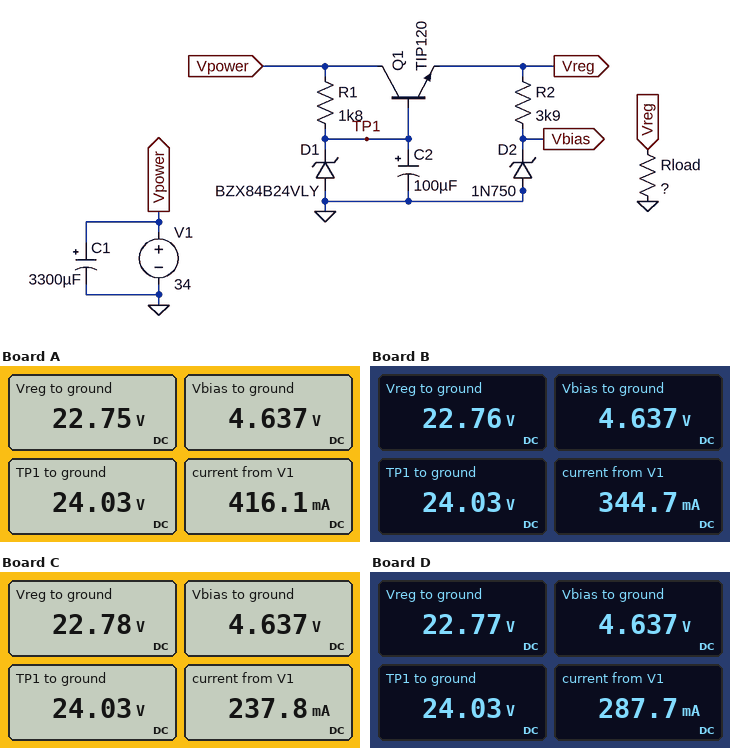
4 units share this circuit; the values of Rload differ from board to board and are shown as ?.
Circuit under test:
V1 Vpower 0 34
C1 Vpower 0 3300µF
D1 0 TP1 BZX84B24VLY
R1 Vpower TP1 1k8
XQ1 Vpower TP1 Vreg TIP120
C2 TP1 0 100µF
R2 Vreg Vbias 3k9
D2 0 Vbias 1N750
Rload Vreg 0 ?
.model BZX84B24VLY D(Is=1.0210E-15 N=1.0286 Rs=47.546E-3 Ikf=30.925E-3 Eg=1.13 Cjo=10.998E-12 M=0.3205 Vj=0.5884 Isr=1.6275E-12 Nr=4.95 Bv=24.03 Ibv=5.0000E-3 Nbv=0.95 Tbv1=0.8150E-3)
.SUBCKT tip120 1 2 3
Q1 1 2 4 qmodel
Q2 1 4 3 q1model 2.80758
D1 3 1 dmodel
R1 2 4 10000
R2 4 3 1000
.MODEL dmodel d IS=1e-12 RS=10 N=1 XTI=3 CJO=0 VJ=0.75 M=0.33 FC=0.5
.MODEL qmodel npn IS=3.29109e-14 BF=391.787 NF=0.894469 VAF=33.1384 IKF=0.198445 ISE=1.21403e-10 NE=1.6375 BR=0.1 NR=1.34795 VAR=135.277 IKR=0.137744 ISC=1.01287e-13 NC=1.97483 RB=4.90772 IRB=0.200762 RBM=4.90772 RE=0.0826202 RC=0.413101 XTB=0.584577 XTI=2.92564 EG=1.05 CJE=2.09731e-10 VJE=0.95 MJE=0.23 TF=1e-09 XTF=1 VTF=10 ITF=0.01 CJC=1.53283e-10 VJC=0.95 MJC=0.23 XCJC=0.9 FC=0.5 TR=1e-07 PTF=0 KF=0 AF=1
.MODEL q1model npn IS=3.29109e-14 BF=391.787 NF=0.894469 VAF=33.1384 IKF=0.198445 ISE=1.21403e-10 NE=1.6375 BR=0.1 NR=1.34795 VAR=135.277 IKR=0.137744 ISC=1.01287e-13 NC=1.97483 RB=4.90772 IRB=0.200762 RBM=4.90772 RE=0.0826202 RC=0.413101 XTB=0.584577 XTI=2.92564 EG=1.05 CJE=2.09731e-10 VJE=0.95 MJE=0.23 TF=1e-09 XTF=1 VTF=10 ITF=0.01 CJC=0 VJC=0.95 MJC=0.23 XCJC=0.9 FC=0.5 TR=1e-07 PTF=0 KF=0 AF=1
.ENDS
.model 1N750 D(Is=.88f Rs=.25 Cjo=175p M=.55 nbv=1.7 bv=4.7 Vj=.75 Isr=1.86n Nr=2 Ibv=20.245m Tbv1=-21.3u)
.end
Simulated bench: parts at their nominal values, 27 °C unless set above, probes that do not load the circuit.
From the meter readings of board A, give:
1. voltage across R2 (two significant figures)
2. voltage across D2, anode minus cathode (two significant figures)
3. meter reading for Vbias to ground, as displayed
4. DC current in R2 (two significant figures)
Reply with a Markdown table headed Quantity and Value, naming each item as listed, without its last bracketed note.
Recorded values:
| Quantity | Value |
|---|---|
| voltage across R2 | 18 V |
| voltage across D2, anode minus cathode | -4.6 V |
| meter reading for Vbias to ground, as displayed | 4.637 V |
| DC current in R2 | 4.6 mA |
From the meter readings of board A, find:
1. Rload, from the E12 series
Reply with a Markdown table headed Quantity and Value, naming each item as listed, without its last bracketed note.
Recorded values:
| Quantity | Value |
|---|---|
| Rload, from the E12 series | 56 Ω |
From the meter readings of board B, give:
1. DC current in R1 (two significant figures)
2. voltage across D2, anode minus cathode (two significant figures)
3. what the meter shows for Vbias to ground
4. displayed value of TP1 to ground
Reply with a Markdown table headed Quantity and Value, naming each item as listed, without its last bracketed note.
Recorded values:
| Quantity | Value |
|---|---|
| DC current in R1 | 5.5 mA |
| voltage across D2, anode minus cathode | -4.6 V |
| what the meter shows for Vbias to ground | 4.637 V |
| displayed value of TP1 to ground | 24.03 V |
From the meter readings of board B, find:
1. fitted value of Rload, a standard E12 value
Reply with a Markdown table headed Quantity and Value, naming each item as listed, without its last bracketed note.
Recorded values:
| Quantity | Value |
|---|---|
| fitted value of Rload, a standard E12 value | 68 Ω |
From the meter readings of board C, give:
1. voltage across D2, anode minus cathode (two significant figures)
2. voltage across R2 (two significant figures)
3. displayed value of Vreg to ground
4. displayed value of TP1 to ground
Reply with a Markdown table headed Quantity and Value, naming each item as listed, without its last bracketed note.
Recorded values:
| Quantity | Value |
|---|---|
| voltage across D2, anode minus cathode | -4.6 V |
| voltage across R2 | 18 V |
| displayed value of Vreg to ground | 22.78 V |
| displayed value of TP1 to ground | 24.03 V |
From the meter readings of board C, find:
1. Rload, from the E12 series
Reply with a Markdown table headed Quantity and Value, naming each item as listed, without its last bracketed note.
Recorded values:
| Quantity | Value |
|---|---|
| Rload, from the E12 series | 100 Ω |
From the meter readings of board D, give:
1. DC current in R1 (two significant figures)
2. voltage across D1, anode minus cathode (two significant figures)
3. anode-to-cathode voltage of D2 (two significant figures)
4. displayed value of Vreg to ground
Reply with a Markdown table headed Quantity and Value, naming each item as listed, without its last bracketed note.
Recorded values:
| Quantity | Value |
|---|---|
| DC current in R1 | 5.5 mA |
| voltage across D1, anode minus cathode | -24 V |
| anode-to-cathode voltage of D2 | -4.6 V |
| displayed value of Vreg to ground | 22.77 V |
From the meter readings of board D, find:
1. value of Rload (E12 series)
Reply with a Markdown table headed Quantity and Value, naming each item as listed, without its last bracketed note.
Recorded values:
| Quantity | Value |
|---|---|
| value of Rload | 82 Ω |
